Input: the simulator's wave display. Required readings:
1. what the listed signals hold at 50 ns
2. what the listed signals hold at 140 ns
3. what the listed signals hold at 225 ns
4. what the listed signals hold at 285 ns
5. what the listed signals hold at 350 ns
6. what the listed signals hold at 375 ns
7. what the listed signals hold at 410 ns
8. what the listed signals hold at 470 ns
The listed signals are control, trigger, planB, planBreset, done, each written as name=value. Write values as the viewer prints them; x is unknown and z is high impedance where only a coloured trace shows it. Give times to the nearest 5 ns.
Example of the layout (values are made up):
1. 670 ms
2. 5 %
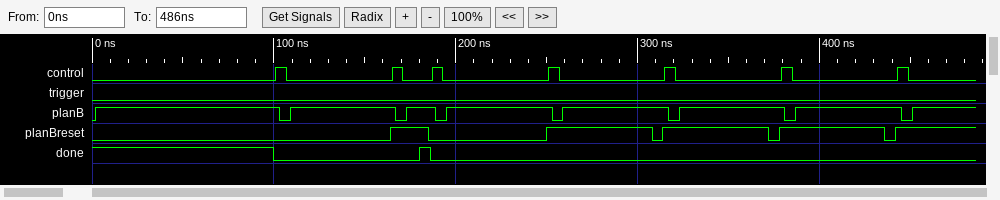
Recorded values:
1. control=0, trigger=0, planB=1, planBreset=0, done=1
2. control=0, trigger=0, planB=1, planBreset=0, done=0
3. control=0, trigger=0, planB=1, planBreset=0, done=0
4. control=0, trigger=0, planB=1, planBreset=1, done=0
5. control=0, trigger=0, planB=1, planBreset=1, done=0
6. control=0, trigger=0, planB=1, planBreset=0, done=0
7. control=0, trigger=0, planB=1, planBreset=1, done=0
8. control=0, trigger=0, planB=1, planBreset=1, done=0
